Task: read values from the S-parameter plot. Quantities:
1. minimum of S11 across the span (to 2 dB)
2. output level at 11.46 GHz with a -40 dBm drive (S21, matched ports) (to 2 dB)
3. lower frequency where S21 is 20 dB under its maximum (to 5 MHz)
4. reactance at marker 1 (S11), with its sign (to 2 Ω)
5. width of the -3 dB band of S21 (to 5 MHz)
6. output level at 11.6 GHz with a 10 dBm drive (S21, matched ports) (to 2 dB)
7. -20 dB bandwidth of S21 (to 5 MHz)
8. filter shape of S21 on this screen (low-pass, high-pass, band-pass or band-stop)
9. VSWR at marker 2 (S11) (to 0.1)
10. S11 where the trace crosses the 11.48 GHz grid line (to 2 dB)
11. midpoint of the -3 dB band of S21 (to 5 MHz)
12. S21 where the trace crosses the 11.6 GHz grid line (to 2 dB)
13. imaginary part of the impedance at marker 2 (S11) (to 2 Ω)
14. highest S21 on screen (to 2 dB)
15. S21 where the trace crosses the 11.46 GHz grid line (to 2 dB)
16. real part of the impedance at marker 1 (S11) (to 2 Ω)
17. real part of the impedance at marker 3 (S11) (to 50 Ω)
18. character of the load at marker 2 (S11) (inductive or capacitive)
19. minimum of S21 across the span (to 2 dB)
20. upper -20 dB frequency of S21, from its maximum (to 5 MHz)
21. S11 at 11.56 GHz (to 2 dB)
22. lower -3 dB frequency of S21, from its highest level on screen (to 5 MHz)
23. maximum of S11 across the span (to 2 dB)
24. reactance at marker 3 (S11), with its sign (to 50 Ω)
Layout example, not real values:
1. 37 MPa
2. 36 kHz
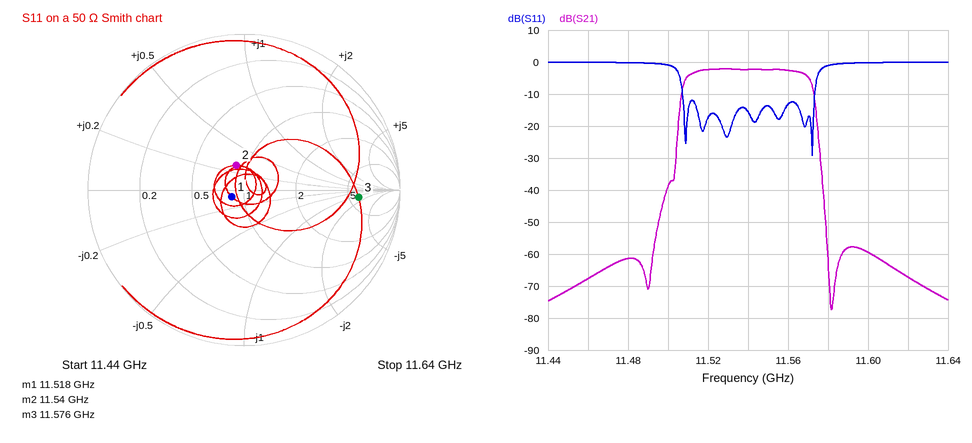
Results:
1. -30 dB
2. -108 dBm
3. 11.505 GHz
4. -4 Ω
5. 60 MHz
6. -50 dBm
7. 70 MHz
8. band-pass
9. 1.4
10. 0 dB
11. 11.540 GHz
12. -60 dB
13. +14 Ω
14. -2 dB
15. -68 dB
16. 42 Ω
17. 300 Ω
18. inductive
19. -78 dB
20. 11.575 GHz
21. -14 dB
22. 11.510 GHz
23. 0 dB
24. -50 Ω
